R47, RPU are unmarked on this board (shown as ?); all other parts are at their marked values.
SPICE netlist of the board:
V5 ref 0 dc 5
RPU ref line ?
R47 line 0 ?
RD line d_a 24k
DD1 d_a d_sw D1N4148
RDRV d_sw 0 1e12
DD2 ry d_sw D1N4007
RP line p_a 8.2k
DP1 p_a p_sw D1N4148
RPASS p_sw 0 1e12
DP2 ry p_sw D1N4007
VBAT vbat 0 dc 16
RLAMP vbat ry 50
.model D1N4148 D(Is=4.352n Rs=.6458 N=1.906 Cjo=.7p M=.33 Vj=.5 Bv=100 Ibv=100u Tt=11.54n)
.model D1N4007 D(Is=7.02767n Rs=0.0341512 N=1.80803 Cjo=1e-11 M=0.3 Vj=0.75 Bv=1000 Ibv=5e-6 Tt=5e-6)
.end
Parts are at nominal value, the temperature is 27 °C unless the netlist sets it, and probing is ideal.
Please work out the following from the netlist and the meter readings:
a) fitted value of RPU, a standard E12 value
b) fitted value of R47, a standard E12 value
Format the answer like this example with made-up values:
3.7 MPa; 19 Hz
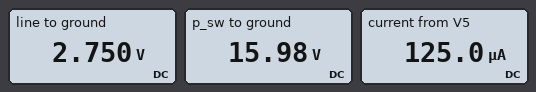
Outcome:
18 kΩ; 22 kΩ
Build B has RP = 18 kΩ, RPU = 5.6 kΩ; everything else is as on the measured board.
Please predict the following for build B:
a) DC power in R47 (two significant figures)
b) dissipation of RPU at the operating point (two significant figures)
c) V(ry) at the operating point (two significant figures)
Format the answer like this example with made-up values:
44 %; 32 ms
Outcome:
720 µW; 180 µW; 16 V
